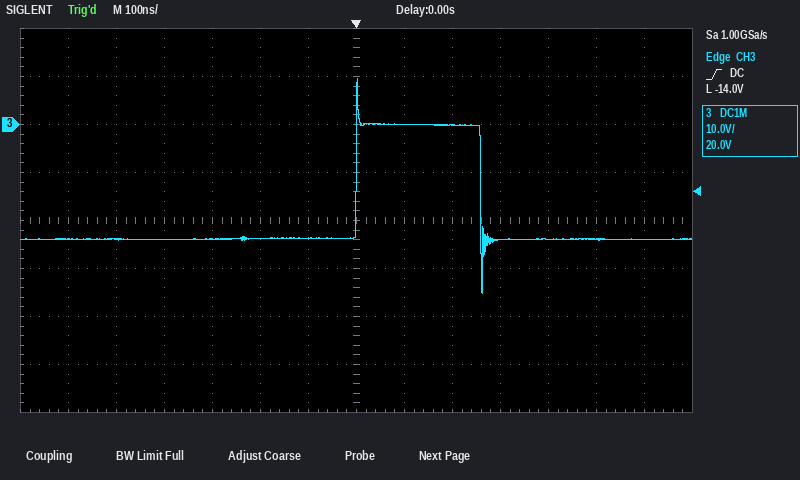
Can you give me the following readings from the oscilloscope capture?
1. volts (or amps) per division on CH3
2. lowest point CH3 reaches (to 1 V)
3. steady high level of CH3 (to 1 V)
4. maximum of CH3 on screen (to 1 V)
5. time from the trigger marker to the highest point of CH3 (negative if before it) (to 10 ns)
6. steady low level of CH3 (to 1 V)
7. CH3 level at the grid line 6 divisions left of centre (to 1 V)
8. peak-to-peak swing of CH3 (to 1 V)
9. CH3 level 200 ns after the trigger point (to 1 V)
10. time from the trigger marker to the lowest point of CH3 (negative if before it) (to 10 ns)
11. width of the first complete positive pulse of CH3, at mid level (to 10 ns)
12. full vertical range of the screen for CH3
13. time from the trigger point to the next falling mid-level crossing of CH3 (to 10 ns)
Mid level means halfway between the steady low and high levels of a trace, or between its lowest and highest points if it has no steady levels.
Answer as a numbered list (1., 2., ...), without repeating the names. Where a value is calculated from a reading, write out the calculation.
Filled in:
1. 10 V
2. -35 V
3. 0 V
4. 10 V
5. 0 ns
6. -24 V
7. -24 V
8. 10 V − (-35 V) = 45 V
9. 0 V
10. +260 ns
11. 260 ns
12. 80 V
13. 260 ns
